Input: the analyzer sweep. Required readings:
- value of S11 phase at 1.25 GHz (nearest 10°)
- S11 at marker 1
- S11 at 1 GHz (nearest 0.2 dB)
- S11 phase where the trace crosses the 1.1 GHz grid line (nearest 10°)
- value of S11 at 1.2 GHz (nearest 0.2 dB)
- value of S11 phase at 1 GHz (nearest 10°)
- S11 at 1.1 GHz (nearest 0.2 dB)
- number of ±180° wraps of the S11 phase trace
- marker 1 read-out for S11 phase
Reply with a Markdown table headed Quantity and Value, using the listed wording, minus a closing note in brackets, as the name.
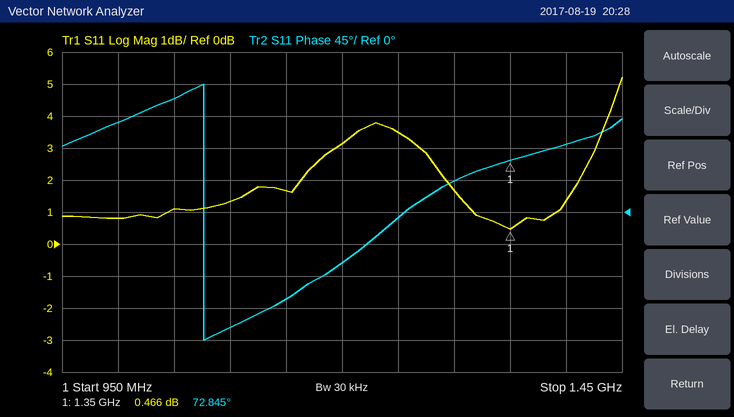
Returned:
| Quantity | Value |
|---|---|
| value of S11 phase at 1.25 GHz | -10° |
| S11 at marker 1 | 0.466 dB |
| S11 at 1 GHz | 0.8 dB |
| S11 phase where the trace crosses the 1.1 GHz grid line | -160° |
| value of S11 at 1.2 GHz | 3.2 dB |
| value of S11 phase at 1 GHz | 130° |
| S11 at 1.1 GHz | 1.4 dB |
| number of ±180° wraps of the S11 phase trace | 1 |
| marker 1 read-out for S11 phase | 72.845° |
